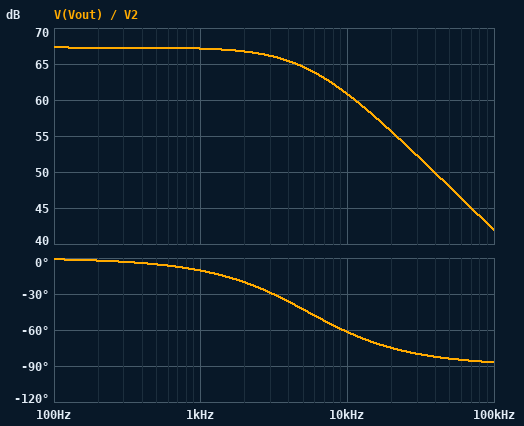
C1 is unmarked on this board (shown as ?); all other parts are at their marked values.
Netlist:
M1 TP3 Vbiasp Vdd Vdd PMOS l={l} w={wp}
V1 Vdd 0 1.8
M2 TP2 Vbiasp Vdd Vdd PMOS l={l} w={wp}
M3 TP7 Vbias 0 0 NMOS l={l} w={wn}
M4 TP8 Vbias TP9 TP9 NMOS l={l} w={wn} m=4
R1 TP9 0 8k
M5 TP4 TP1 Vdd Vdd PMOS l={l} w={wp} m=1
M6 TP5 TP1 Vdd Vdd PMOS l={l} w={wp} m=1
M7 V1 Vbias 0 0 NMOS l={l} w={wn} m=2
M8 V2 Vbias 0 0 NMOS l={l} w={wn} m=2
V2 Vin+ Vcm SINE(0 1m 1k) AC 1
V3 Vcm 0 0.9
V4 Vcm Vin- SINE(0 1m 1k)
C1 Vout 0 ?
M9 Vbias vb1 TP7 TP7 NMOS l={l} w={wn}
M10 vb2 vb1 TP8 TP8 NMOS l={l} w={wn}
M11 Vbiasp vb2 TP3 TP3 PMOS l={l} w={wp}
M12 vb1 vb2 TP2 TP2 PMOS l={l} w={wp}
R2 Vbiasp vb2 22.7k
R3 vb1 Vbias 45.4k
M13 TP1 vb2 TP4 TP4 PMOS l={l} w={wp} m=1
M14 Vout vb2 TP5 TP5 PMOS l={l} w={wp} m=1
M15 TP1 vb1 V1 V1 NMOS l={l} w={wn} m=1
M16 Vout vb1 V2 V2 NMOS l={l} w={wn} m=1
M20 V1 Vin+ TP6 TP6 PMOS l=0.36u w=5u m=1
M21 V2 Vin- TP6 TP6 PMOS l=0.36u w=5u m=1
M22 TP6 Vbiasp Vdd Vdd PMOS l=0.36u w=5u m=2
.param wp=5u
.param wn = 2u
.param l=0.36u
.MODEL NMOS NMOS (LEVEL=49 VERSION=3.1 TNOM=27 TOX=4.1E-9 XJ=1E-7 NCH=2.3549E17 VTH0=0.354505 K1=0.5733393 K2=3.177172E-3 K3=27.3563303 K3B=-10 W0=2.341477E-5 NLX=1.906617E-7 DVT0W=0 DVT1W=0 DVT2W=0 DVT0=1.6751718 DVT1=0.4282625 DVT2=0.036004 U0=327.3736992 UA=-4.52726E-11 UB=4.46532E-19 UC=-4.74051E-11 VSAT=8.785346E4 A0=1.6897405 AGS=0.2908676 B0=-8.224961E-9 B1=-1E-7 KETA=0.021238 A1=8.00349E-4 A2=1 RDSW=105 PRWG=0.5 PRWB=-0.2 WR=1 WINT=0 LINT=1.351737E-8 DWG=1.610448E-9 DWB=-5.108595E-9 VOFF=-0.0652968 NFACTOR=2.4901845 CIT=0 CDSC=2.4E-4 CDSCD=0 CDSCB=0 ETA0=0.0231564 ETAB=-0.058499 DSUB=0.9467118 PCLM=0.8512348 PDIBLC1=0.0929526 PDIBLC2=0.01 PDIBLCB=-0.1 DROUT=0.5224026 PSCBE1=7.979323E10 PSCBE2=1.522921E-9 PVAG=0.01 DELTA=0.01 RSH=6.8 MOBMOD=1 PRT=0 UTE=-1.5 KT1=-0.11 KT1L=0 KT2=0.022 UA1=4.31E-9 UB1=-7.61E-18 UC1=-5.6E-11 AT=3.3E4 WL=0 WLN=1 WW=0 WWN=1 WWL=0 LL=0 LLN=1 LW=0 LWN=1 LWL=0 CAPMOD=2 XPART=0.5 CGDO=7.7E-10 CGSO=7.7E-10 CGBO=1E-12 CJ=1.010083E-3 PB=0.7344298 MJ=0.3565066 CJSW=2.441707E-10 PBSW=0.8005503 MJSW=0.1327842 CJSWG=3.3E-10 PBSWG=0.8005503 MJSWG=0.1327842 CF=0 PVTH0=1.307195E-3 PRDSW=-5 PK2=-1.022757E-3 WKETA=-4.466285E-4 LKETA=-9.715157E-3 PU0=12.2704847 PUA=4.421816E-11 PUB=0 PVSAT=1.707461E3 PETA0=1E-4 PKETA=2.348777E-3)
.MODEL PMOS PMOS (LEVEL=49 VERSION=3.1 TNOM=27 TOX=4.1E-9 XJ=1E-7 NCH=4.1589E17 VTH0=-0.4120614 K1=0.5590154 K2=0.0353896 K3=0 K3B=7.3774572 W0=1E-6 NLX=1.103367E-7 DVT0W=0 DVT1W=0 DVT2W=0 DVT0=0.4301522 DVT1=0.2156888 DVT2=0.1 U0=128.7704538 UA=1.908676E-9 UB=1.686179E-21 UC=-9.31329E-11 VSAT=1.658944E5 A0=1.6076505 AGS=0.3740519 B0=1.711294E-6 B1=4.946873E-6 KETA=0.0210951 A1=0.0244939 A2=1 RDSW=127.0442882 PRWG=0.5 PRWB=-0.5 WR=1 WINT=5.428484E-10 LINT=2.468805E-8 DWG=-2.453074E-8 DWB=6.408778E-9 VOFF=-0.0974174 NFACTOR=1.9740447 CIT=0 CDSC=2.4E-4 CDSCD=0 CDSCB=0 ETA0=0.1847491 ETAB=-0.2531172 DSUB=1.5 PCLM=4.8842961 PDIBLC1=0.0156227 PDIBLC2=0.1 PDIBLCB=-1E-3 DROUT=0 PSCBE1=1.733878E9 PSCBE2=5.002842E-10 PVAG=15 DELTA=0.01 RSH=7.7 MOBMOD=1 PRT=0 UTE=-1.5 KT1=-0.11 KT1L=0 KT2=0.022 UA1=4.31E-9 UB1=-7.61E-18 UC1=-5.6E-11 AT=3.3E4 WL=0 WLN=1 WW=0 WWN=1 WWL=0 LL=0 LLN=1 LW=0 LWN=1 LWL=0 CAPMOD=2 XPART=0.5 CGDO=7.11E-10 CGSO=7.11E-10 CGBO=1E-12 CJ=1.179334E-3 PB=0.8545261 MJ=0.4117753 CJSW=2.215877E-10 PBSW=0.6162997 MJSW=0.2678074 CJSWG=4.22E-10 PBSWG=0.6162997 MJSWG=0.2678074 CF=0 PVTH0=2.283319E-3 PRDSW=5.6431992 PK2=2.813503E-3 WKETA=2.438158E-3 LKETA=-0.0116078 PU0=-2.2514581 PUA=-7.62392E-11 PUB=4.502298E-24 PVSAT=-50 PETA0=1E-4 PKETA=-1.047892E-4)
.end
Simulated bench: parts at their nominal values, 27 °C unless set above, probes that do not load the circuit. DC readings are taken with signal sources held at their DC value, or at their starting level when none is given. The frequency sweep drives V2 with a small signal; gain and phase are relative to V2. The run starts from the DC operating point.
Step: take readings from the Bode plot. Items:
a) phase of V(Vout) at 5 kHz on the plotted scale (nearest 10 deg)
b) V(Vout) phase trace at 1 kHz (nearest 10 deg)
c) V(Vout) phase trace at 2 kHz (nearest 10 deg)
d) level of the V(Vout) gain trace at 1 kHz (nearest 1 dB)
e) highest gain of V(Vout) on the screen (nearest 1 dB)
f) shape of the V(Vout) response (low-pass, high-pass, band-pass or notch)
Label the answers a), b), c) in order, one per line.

a) -40 deg
b) -10 deg
c) -20 deg
d) 67 dB
e) 67 dB
f) low-pass
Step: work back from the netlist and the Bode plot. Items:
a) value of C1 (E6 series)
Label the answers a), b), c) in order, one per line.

a) 1.5 pF
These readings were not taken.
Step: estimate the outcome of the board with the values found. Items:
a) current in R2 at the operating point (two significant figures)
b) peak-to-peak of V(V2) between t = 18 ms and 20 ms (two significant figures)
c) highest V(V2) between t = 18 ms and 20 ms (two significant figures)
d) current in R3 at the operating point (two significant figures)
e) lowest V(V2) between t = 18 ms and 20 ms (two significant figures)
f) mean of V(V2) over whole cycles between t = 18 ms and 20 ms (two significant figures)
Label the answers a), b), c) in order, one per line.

a) 9.0 µA
b) 60 mV
c) 420 mV
d) 9.0 µA
e) 360 mV
f) 400 mV
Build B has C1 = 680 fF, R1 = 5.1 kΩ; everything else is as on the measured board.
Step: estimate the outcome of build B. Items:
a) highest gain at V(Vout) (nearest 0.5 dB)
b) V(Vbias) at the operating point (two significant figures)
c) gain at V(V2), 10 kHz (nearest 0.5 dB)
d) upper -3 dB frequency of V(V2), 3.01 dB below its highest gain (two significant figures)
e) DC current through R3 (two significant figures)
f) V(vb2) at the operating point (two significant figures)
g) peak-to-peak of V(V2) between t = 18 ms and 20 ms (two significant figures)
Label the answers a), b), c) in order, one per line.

a) 64.5 dB
b) 640 mV
c) 25.5 dB
d) 23 kHz
e) 16 µA
f) 770 mV
g) 62 mV
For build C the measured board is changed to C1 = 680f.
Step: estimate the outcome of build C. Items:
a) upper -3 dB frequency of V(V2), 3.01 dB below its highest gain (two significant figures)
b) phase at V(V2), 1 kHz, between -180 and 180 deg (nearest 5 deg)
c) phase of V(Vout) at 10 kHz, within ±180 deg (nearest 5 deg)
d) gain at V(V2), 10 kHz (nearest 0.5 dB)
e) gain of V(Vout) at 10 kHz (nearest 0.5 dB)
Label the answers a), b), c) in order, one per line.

a) 12 kHz
b) -5 deg
c) -40 deg
d) 23.5 dB
e) 65.0 dB
